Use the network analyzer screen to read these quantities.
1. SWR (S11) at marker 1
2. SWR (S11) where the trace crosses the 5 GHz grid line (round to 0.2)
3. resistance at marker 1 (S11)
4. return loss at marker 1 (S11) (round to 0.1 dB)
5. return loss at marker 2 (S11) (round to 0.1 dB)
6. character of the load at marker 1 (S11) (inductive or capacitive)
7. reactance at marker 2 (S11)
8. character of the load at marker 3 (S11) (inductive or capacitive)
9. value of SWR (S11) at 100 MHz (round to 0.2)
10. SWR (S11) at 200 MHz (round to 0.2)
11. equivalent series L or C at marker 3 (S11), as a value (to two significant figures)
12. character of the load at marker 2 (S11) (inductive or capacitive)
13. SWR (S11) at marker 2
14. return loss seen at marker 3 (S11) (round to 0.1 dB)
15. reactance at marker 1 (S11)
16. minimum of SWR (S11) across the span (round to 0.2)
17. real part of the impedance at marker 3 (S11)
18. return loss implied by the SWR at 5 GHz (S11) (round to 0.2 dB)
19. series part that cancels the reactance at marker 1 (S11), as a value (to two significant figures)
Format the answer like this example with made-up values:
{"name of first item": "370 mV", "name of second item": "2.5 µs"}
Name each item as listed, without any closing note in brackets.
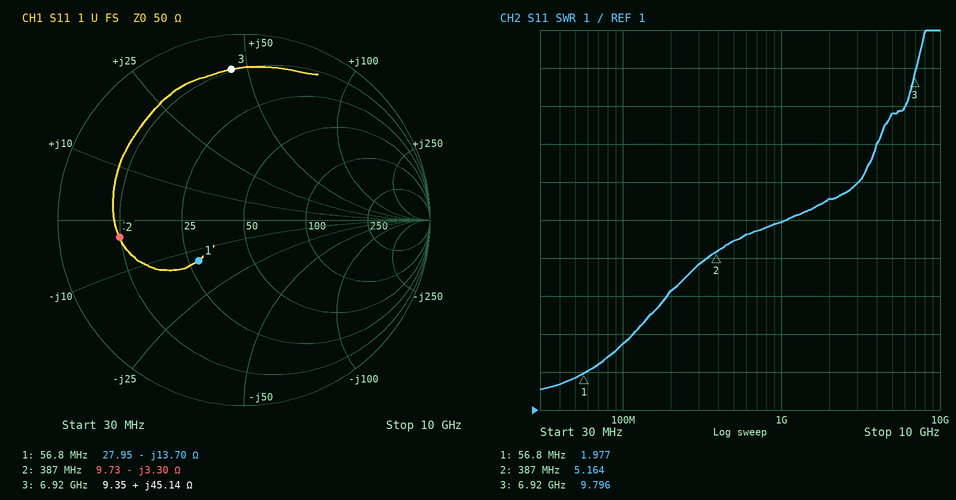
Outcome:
{"SWR (S11) at marker 1": "1.977", "SWR (S11) where the trace crosses the 5 GHz grid line": "8.8", "resistance at marker 1": "27.95 Ω", "return loss at marker 1 (S11)": "9.7 dB", "return loss at marker 2 (S11)": "3.4 dB", "character of the load at marker 1 (S11)": "capacitive", "reactance at marker 2": "-3.30 Ω", "character of the load at marker 3 (S11)": "inductive", "value of SWR (S11) at 100 MHz": "2.8", "SWR (S11) at 200 MHz": "4.2", "equivalent series L or C at marker 3 (S11), as a value": "1.0 nH", "character of the load at marker 2 (S11)": "capacitive", "SWR (S11) at marker 2": "5.164", "return loss seen at marker 3 (S11)": "1.8 dB", "reactance at marker 1": "-13.70 Ω", "minimum of SWR (S11) across the span": "1.6", "real part of the impedance at marker 3": "9.35 Ω", "return loss implied by the SWR at 5 GHz (S11)": "2.0 dB", "series part that cancels the reactance at marker 1 (S11), as a value": "38 nH"}
